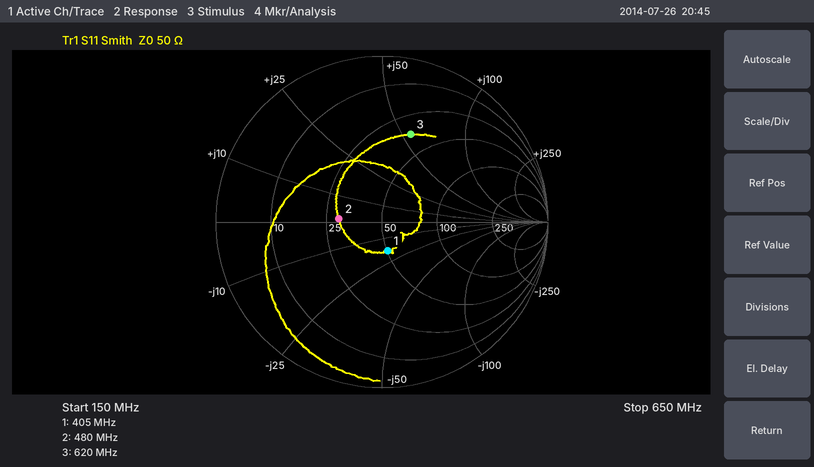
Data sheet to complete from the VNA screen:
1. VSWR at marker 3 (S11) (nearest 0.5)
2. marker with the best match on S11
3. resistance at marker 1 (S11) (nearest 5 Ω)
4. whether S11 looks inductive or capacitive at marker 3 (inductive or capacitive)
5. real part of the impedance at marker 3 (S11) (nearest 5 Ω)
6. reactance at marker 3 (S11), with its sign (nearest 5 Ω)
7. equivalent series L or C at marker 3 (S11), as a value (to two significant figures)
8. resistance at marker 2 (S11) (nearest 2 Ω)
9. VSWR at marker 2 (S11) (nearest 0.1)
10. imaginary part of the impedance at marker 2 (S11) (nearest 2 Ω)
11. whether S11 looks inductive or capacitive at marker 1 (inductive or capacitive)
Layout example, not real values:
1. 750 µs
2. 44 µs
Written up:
1. 3.5
2. marker 1
3. 50 Ω
4. inductive
5. 35 Ω
6. +55 Ω
7. 14 nH
8. 30 Ω
9. 1.7
10. +2 Ω
11. capacitive
